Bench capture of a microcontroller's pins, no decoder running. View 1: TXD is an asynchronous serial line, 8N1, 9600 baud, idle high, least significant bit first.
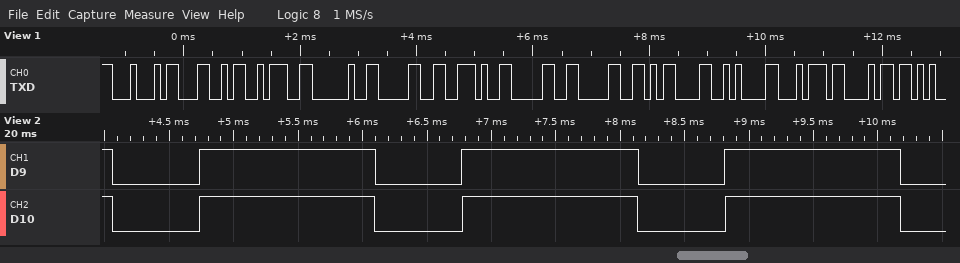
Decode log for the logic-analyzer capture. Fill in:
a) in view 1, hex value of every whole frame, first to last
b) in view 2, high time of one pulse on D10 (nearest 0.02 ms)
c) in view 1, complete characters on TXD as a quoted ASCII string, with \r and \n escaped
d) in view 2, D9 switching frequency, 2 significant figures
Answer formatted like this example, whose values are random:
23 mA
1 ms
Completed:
44 4C 3A 20 30 2E 30 30 0D 0A 74 68
1.36 ms
"DL: 0.00\r\nth"
490 Hz
